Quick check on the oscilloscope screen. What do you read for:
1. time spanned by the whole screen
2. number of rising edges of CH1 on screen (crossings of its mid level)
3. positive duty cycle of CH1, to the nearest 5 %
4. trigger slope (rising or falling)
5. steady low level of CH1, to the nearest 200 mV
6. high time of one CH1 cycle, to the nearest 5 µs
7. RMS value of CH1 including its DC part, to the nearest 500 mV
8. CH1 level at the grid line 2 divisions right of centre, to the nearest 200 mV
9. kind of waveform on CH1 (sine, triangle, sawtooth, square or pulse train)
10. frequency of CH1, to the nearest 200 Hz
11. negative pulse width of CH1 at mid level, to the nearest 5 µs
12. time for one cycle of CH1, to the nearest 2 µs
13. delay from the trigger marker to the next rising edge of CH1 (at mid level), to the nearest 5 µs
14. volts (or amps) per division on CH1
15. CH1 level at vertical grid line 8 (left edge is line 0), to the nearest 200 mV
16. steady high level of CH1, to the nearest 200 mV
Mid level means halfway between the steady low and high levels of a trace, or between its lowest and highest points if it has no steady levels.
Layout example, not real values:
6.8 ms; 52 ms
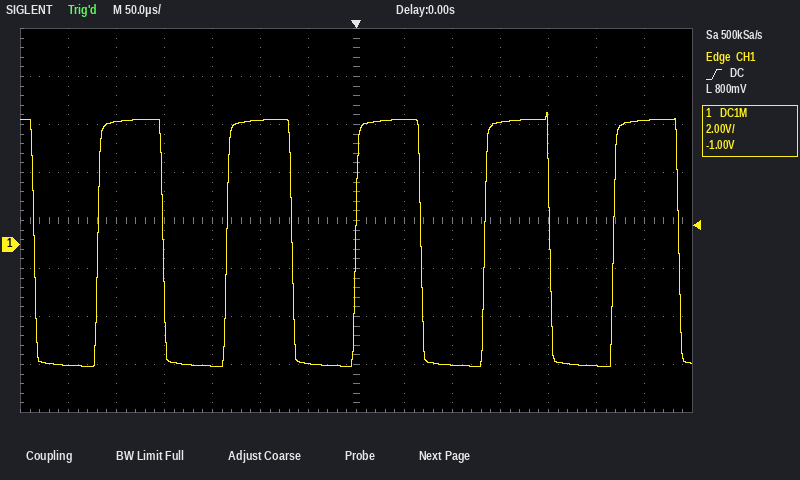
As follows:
700 µs; 5; 50 %; rising; -5.0 V; 70 µs; 5.0 V; -5.0 V; square; 7.4 kHz; 65 µs; 134 µs; 135 µs; 2 V; 5.2 V; 5.2 V
